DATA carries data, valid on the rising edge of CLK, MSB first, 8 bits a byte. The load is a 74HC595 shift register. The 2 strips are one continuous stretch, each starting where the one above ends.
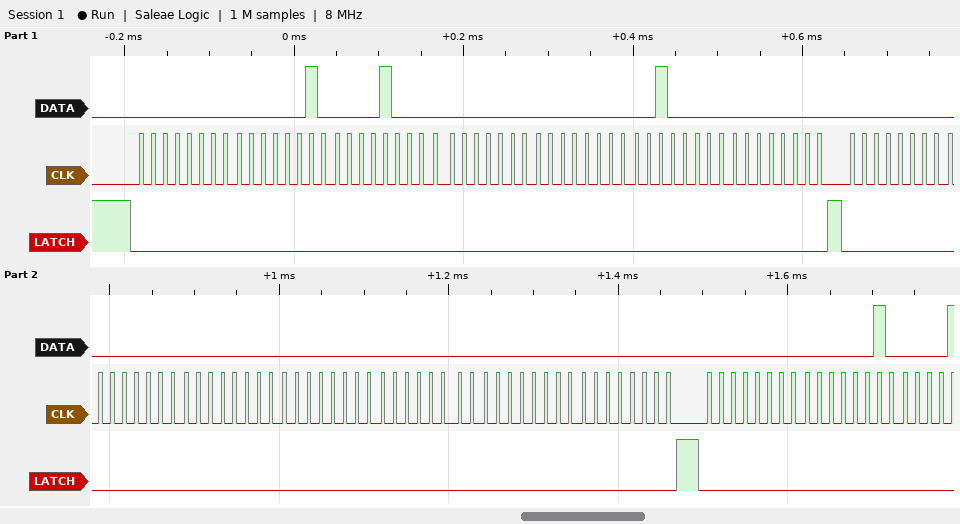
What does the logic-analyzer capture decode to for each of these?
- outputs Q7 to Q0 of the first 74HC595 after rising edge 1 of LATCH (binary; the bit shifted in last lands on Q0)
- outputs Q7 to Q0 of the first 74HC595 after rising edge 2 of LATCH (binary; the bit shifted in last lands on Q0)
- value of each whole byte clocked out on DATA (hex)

00000000
00000000
00 02 08 00 00 20 00 00 00 00 00 00 00 00 00 02
